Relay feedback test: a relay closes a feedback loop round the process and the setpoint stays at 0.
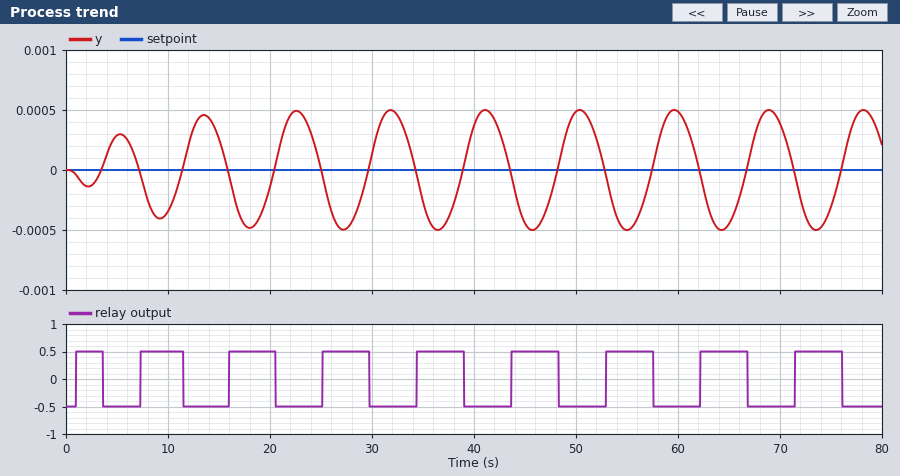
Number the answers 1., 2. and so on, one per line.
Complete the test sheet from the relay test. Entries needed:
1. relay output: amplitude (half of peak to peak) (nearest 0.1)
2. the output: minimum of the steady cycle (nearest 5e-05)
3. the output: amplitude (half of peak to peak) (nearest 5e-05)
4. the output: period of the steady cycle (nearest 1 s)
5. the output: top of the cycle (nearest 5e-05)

1. 0.5
2. -0.00050
3. 0.00050
4. 9 s
5. 0.00050
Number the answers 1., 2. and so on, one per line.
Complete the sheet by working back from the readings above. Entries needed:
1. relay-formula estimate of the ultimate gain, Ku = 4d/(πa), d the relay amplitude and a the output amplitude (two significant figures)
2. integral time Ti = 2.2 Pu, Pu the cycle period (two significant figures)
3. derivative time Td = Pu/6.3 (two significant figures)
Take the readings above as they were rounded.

1. 1300
2. 20 s
3. 1.4 s
